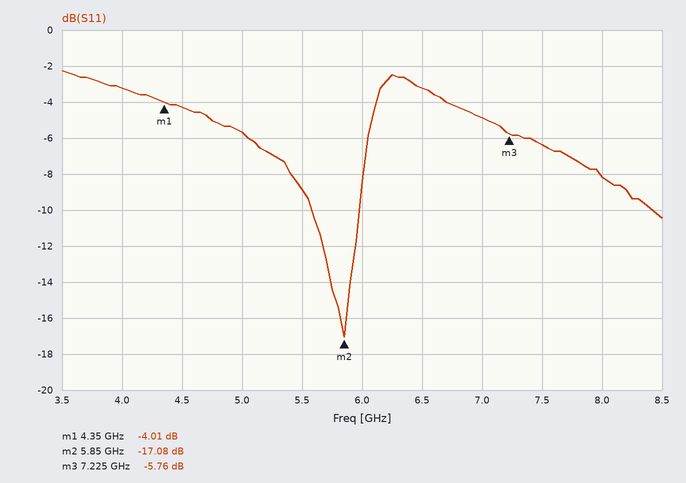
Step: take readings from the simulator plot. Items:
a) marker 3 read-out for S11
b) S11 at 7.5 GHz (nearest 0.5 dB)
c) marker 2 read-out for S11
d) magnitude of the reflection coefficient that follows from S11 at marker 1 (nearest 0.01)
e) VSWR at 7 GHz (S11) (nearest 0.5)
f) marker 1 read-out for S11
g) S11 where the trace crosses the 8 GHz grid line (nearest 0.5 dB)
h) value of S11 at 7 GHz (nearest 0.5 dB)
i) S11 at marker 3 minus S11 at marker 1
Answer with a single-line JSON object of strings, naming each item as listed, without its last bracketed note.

{"marker 3 read-out for S11": "-5.76 dB", "S11 at 7.5 GHz": "-6.5 dB", "marker 2 read-out for S11": "-17.08 dB", "magnitude of the reflection coefficient that follows from S11 at marker 1": "0.63", "VSWR at 7 GHz (S11)": "3.5", "marker 1 read-out for S11": "-4.01 dB", "S11 where the trace crosses the 8 GHz grid line": "-8.0 dB", "value of S11 at 7 GHz": "-5.0 dB", "S11 at marker 3 minus S11 at marker 1": "-1.75 dB"}
